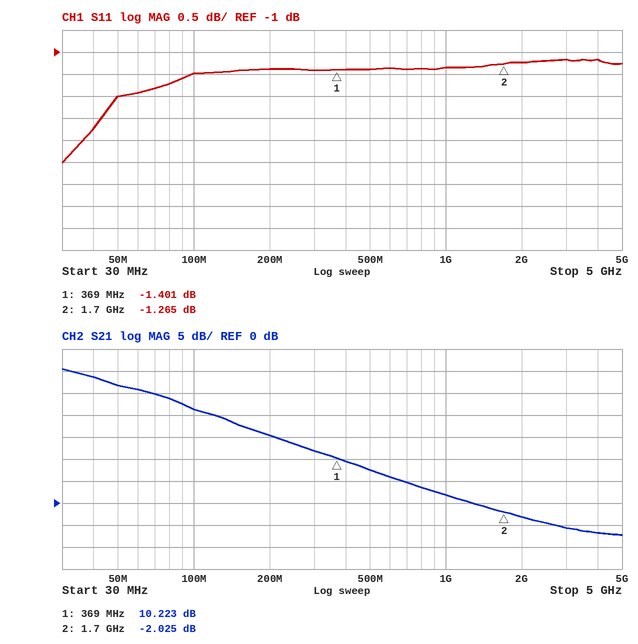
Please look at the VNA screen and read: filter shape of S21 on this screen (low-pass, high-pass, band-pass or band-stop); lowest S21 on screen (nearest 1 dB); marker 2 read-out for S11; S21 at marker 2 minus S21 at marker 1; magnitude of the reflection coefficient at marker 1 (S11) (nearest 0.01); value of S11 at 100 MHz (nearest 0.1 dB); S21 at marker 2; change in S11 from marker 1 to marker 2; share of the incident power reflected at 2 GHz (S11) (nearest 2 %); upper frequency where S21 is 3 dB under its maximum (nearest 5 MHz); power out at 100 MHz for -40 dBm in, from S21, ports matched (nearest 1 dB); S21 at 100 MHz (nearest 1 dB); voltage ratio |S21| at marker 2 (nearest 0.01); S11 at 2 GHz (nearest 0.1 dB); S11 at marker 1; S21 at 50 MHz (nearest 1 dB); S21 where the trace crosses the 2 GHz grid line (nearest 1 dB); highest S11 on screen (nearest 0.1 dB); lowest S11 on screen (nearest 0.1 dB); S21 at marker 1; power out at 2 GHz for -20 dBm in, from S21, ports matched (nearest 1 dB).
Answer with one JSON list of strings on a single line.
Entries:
["low-pass", "-7 dB", "-1.265 dB", "-12.248 dB", "0.85", "-1.5 dB", "-2.025 dB", "0.136 dB", "76 %", "45 MHz", "-19 dBm", "21 dB", "0.79", "-1.2 dB", "-1.401 dB", "27 dB", "-3 dB", "-1.2 dB", "-3.5 dB", "10.223 dB", "-23 dBm"]
